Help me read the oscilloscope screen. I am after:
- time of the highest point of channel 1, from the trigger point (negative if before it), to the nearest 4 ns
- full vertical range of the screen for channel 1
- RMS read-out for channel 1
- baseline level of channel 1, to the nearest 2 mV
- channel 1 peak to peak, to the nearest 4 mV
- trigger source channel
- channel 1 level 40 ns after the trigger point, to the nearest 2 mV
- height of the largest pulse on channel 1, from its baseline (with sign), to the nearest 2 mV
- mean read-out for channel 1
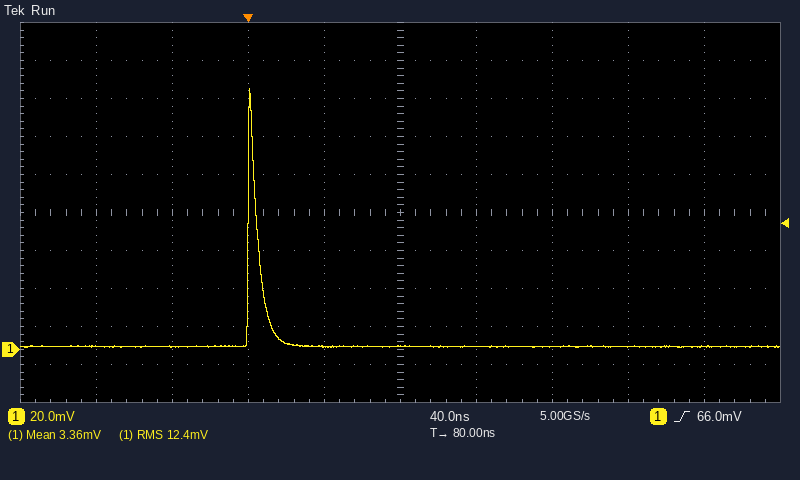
0 ns
200 mV
12.4 mV
2 mV
136 mV
channel 1
2 mV
+136 mV
3.36 mV
